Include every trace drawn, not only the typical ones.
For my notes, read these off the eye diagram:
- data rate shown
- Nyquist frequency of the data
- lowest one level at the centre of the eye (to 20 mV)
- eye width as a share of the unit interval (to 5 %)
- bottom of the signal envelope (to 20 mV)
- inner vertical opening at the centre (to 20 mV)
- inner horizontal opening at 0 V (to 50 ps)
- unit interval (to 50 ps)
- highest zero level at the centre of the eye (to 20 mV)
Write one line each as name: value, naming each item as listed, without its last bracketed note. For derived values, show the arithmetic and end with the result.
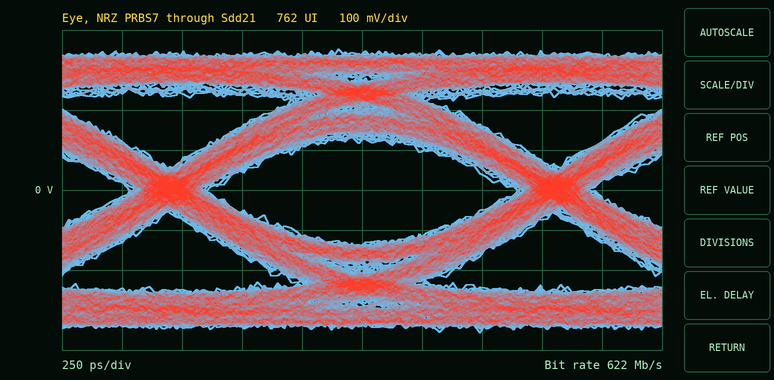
data rate shown: 622 Mb/s
Nyquist frequency of the data: 311 MHz
lowest one level at the centre of the eye: 120 mV
eye width as a share of the unit interval: 1.30 ns / 1.60 ns ≈ 81.2 %, so 80 % to the nearest 5 %
bottom of the signal envelope: -360 mV
inner vertical opening at the centre: 260 mV
inner horizontal opening at 0 V: 1.30 ns
unit interval: 1.60 ns
highest zero level at the centre of the eye: -140 mV
